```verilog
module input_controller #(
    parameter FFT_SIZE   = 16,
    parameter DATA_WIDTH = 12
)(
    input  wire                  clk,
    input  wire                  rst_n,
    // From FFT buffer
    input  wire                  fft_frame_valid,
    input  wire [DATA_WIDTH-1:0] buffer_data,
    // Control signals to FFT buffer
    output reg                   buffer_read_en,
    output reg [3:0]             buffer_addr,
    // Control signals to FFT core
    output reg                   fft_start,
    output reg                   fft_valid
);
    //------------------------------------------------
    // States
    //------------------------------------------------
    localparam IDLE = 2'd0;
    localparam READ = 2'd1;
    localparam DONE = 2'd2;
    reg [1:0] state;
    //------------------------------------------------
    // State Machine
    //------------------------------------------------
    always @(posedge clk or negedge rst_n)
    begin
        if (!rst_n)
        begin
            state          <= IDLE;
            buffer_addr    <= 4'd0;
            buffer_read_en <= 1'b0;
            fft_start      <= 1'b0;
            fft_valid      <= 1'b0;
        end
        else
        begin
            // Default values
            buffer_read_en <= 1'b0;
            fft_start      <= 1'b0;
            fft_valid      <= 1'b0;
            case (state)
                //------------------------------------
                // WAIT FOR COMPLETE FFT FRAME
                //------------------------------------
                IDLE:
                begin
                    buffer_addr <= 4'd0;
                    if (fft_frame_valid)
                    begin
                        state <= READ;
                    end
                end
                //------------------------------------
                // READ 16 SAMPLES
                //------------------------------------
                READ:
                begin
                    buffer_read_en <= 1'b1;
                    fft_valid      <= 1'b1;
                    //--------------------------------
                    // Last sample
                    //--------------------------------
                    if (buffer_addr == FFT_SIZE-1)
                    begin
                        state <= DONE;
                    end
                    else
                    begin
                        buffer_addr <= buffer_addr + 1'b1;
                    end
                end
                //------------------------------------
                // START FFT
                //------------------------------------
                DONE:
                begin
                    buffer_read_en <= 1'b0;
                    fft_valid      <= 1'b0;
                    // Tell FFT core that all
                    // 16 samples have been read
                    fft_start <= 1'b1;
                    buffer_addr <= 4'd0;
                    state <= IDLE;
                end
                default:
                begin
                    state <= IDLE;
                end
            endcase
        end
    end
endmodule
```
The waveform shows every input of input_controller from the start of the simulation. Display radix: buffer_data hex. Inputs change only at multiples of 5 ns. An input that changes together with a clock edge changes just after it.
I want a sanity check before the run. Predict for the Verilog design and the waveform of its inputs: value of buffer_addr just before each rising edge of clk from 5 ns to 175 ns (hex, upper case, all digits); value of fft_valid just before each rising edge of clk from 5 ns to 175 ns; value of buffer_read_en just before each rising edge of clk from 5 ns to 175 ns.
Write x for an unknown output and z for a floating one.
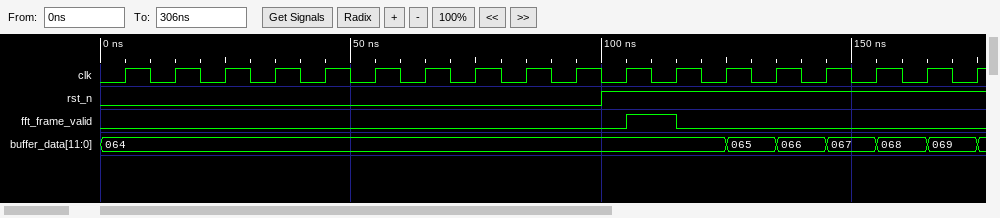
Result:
0, 0, 0, 0, 0, 0, 0, 0, 0, 0, 0, 0, 0, 1, 2, 3, 4, 5
0 0 0 0 0 0 0 0 0 0 0 0 0 1 1 1 1 1
0 0 0 0 0 0 0 0 0 0 0 0 0 1 1 1 1 1
